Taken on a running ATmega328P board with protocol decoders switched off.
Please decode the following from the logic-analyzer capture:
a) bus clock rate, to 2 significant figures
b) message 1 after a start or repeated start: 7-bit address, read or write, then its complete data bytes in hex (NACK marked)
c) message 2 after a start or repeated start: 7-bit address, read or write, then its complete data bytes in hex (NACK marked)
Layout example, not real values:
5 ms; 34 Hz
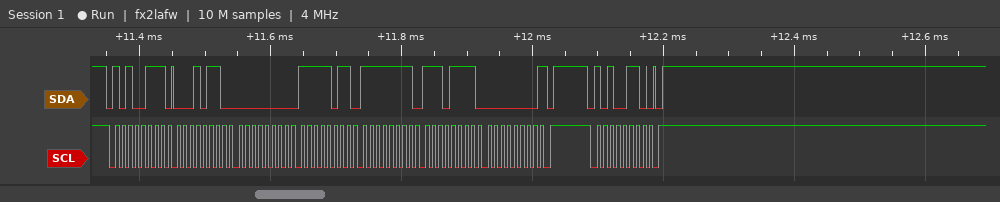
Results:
100 kHz; 0x53 read: 16 00 FB FF EF 00 NACK; 0x53 write
